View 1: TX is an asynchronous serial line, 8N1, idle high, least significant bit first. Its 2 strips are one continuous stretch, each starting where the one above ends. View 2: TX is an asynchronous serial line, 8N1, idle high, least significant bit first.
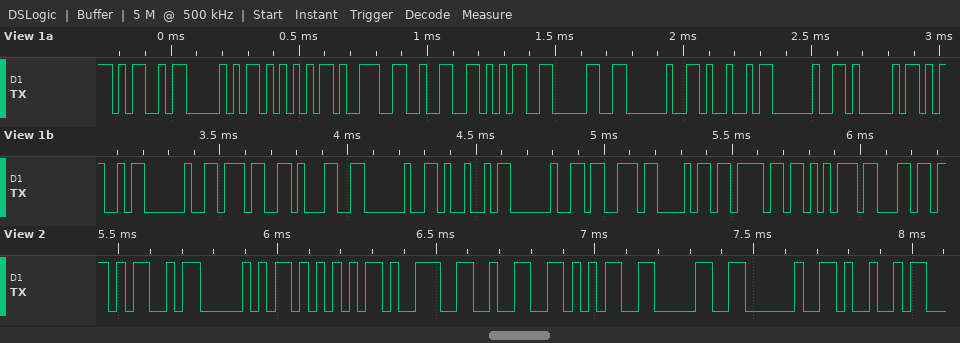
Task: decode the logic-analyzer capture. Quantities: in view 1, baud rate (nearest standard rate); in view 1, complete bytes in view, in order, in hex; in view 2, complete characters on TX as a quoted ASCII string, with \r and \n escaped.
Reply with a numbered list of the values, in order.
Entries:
1. 38400 baud
2. 4D 50 55 39 32 35 30 20 49 20 41 4D 20 37 31 20 49 20 73 68 6F 75 6C
3. "MPU9250 I"
